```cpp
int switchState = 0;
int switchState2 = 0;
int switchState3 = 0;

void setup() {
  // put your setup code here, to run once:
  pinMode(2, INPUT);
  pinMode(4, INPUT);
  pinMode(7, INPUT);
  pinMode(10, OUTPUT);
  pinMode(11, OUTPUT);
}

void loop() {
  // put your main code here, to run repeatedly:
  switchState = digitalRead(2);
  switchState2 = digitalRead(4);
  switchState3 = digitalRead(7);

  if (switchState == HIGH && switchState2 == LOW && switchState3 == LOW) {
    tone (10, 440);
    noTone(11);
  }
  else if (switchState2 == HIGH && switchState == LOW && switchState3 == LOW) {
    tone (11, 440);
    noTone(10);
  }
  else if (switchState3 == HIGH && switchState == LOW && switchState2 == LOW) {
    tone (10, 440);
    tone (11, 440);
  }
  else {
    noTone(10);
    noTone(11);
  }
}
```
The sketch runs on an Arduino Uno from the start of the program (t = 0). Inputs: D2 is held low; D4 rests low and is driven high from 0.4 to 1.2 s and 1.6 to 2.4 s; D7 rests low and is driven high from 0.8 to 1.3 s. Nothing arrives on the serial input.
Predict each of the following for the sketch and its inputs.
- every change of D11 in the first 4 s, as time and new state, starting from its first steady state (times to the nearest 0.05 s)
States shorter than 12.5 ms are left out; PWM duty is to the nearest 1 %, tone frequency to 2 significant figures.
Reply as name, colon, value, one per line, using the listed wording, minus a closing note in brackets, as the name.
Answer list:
every change of D11 in the first 4 s, as time and new state, starting from its first steady state: 0 s low; 0.4 s tone 440 Hz; 0.8 s low; 1.6 s tone 440 Hz; 2.4 s low
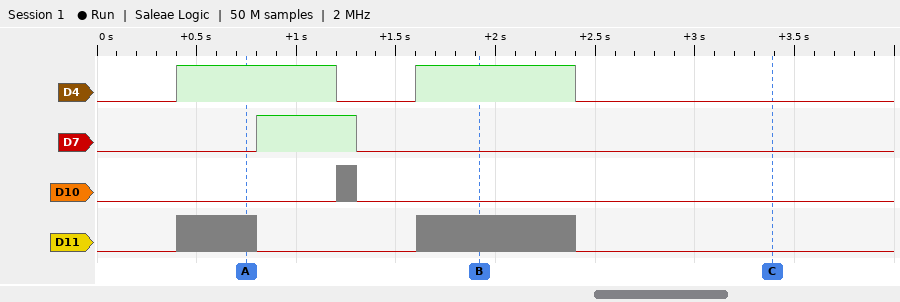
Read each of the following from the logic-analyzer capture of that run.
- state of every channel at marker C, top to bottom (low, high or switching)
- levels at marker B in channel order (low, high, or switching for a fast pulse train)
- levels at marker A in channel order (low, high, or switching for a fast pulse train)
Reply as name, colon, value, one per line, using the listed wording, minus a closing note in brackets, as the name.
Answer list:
state of every channel at marker C, top to bottom: D4 low, D7 low, D10 low, D11 low
levels at marker B in channel order: D4 high, D7 low, D10 low, D11 switching
levels at marker A in channel order: D4 high, D7 low, D10 low, D11 switching
